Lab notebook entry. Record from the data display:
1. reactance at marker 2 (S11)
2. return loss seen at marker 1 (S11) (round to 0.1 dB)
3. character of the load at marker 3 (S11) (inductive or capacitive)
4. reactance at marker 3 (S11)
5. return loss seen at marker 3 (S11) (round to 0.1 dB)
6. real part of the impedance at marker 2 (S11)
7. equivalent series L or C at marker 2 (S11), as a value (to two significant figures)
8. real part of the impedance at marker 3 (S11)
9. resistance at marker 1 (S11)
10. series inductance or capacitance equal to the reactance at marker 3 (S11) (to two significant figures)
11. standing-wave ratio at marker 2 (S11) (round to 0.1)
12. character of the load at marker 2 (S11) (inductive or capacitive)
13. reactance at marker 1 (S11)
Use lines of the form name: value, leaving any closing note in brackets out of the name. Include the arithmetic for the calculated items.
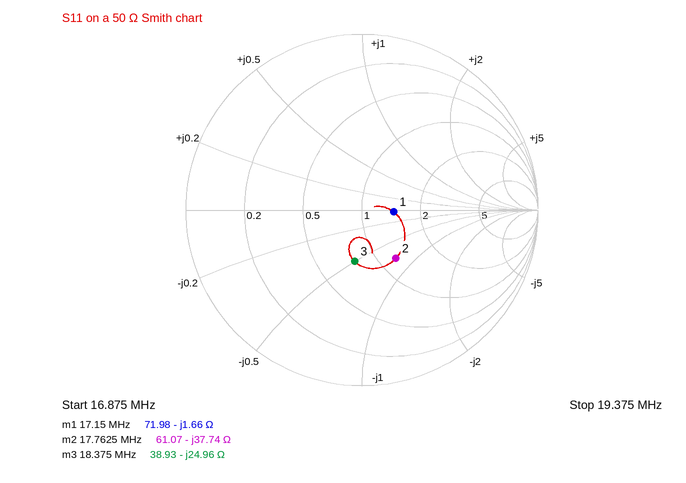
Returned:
reactance at marker 2: -37.74 Ω
return loss seen at marker 1 (S11): 14.9 dB
character of the load at marker 3 (S11): capacitive
reactance at marker 3: -24.96 Ω
return loss seen at marker 3 (S11): 10.6 dB
real part of the impedance at marker 2: 61.07 Ω
equivalent series L or C at marker 2 (S11), as a value: C = 1/(2π × 17.7625 MHz × 37.74 Ω) ≈ 237 pF, so 240 pF to two significant figures
real part of the impedance at marker 3: 38.93 Ω
resistance at marker 1: 71.98 Ω
series inductance or capacitance equal to the reactance at marker 3 (S11): C = 1/(2π × 18.375 MHz × 24.96 Ω) ≈ 347 pF, so 350 pF to two significant figures
standing-wave ratio at marker 2 (S11): 2.0
character of the load at marker 2 (S11): capacitive
reactance at marker 1: -1.66 Ω
